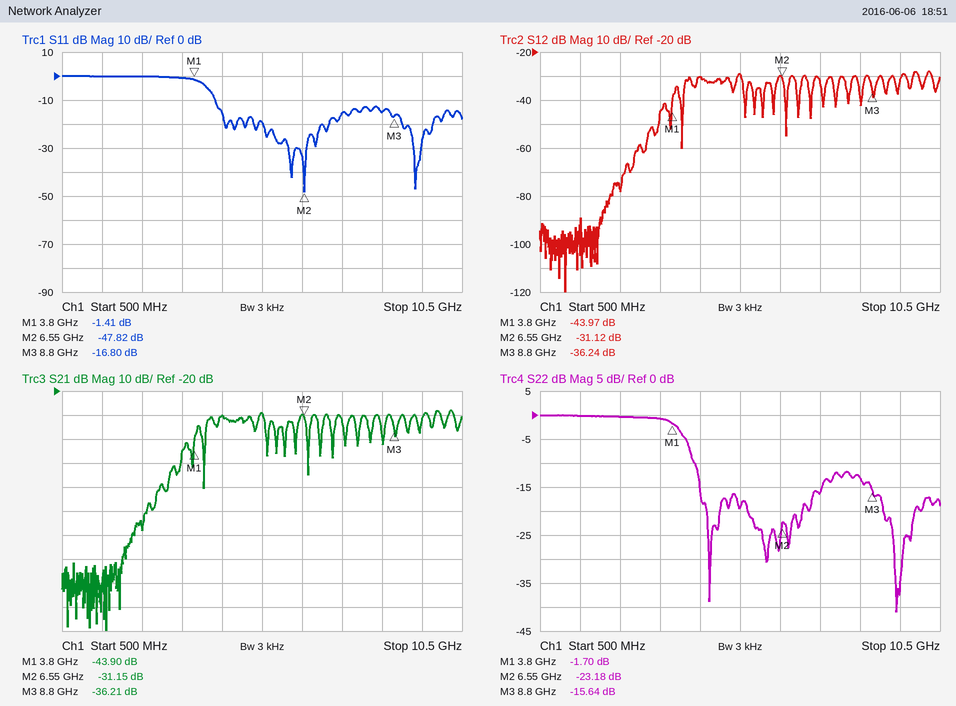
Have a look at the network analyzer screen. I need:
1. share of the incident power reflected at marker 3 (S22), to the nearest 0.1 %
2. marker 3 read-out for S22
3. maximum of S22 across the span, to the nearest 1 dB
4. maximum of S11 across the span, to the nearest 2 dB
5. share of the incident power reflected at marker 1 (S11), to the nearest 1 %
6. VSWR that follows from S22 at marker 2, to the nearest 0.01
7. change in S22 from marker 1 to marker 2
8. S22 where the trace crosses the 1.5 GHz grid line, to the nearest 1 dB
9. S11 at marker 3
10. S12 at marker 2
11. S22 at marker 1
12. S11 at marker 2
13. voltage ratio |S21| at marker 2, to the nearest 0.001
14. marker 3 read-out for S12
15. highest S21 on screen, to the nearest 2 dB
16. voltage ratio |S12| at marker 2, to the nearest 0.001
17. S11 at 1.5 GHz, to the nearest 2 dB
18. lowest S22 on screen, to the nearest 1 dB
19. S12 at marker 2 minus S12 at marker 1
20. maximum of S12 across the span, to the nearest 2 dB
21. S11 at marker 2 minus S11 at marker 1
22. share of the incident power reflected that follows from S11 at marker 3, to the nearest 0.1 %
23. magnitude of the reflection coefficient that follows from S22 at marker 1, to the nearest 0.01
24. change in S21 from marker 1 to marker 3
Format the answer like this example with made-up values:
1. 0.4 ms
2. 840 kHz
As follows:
1. 2.7 %
2. -15.64 dB
3. 0 dB
4. 0 dB
5. 72 %
6. 1.15
7. -21.48 dB
8. 0 dB
9. -16.80 dB
10. -31.12 dB
11. -1.70 dB
12. -47.82 dB
13. 0.028
14. -36.24 dB
15. -28 dB
16. 0.028
17. 0 dB
18. -41 dB
19. 12.85 dB
20. -28 dB
21. -46.41 dB
22. 2.1 %
23. 0.82
24. 7.69 dB
